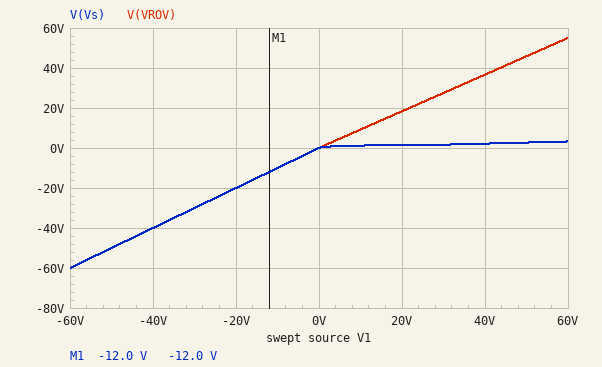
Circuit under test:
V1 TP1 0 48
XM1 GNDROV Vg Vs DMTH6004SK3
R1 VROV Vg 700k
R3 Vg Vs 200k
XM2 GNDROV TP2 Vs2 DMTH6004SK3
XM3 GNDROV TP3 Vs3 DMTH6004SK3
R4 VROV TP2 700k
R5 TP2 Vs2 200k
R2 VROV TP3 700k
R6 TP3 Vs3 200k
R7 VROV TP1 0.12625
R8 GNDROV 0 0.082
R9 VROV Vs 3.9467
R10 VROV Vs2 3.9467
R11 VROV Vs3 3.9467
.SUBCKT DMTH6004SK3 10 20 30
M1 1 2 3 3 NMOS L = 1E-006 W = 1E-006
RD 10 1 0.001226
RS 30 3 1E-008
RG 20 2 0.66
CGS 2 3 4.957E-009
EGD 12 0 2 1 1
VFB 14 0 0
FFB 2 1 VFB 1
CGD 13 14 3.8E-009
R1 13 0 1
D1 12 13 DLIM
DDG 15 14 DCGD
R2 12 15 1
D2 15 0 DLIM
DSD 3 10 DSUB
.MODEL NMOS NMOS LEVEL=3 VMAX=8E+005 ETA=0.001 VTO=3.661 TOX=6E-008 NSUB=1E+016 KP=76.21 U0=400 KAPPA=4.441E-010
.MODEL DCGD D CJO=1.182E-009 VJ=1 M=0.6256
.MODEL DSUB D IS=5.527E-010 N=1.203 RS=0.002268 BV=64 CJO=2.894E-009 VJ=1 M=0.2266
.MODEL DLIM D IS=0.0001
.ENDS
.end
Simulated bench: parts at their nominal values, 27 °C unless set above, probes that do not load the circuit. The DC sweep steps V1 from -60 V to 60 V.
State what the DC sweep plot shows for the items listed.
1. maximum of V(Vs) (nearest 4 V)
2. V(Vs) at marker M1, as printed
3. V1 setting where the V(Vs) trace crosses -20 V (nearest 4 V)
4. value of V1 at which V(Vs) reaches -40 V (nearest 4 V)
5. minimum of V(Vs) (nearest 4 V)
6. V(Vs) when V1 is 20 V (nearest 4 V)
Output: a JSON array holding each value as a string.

["4 V", "-12.0 V", "-20 V", "-40 V", "-60 V", "0 V"]
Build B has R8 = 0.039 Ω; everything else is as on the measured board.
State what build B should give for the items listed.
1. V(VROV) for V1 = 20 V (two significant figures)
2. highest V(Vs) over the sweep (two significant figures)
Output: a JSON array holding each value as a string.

["18 V", "1.6 V"]
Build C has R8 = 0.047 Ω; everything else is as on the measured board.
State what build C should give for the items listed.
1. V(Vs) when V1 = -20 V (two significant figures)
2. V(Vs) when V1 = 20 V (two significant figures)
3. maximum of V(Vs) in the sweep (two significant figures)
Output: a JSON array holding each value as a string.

["-20 V", "790 mV", "1.9 V"]
